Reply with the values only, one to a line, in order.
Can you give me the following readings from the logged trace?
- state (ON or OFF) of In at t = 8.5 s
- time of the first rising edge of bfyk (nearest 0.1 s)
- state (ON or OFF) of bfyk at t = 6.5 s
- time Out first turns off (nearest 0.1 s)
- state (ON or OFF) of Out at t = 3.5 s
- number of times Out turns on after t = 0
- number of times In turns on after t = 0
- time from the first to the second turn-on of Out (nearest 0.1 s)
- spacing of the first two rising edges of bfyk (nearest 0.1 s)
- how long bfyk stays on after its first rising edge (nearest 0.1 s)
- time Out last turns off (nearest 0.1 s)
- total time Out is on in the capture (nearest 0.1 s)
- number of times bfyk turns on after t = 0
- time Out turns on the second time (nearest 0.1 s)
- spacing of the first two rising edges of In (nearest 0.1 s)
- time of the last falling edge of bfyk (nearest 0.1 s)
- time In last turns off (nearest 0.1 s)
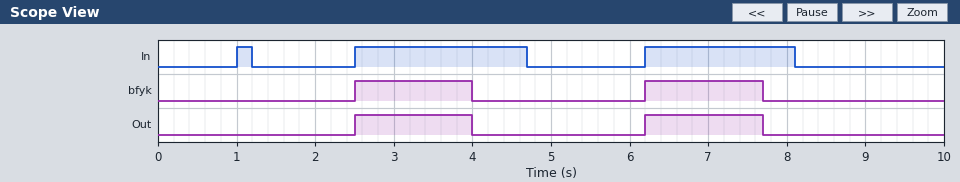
OFF
2.5 s
ON
4.0 s
ON
2
3
3.7 s
3.7 s
1.5 s
7.7 s
3.0 s
2
6.2 s
1.5 s
7.7 s
8.1 s
